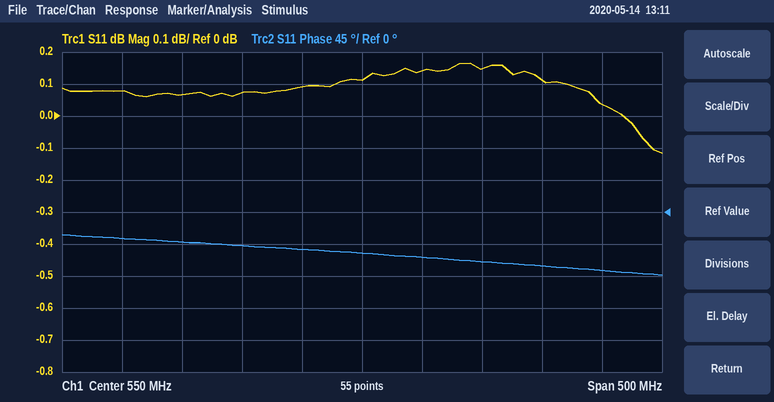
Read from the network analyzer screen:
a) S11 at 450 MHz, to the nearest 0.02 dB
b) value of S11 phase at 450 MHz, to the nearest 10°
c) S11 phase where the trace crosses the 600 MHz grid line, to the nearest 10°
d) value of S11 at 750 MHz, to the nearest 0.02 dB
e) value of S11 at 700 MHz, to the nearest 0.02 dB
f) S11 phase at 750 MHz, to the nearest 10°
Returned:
0.08 dB
-50°
-60°
0.04 dB
0.12 dB
-80°
